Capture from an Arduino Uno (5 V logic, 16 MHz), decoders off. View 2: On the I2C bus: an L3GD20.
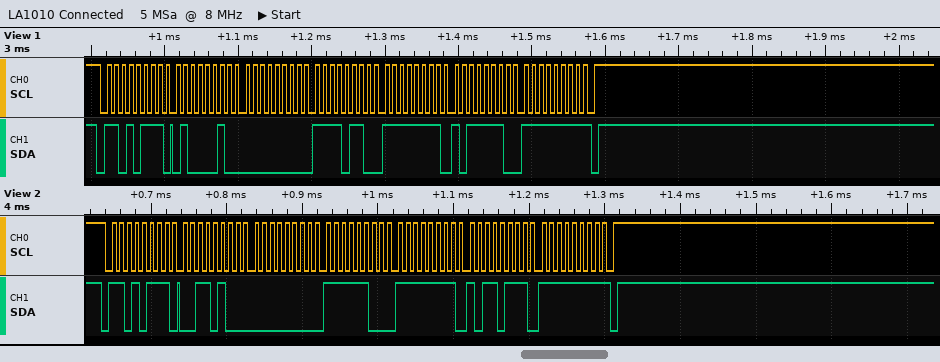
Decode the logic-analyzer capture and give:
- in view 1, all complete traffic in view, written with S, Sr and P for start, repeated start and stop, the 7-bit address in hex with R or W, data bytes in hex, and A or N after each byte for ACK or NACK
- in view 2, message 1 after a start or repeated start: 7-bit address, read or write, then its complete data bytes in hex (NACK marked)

S 6BR A 42 A 00 A F6 A FF A BE A FF N P
0x6B read: 34 00 FC FF B7 FF NACK
